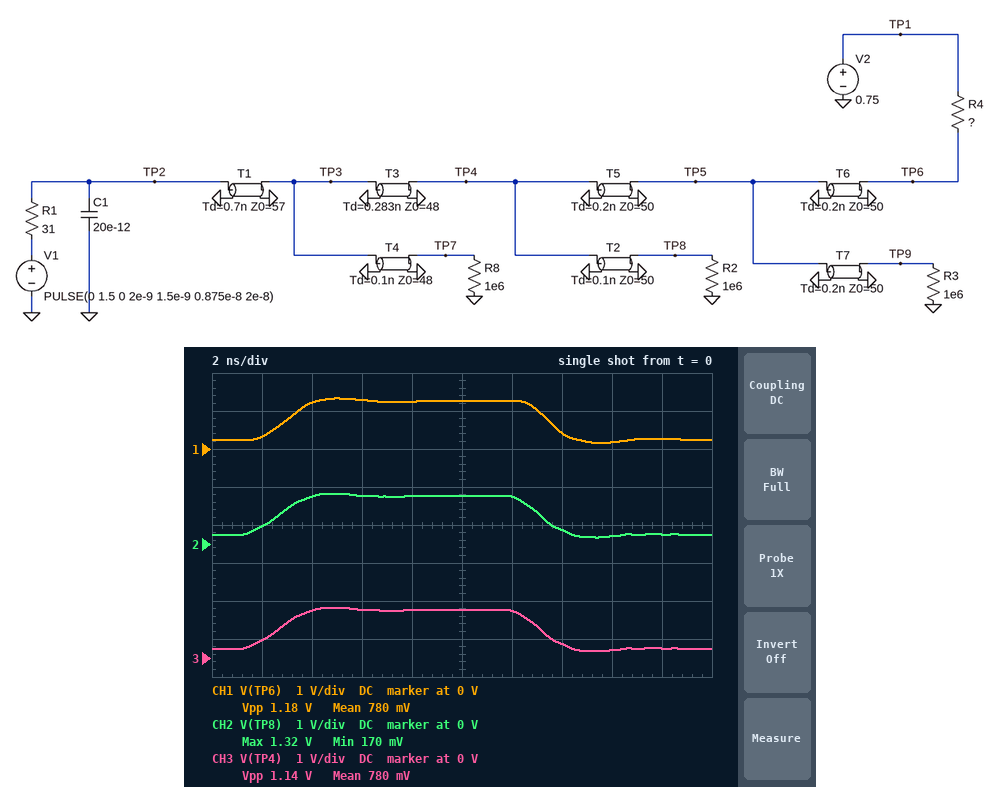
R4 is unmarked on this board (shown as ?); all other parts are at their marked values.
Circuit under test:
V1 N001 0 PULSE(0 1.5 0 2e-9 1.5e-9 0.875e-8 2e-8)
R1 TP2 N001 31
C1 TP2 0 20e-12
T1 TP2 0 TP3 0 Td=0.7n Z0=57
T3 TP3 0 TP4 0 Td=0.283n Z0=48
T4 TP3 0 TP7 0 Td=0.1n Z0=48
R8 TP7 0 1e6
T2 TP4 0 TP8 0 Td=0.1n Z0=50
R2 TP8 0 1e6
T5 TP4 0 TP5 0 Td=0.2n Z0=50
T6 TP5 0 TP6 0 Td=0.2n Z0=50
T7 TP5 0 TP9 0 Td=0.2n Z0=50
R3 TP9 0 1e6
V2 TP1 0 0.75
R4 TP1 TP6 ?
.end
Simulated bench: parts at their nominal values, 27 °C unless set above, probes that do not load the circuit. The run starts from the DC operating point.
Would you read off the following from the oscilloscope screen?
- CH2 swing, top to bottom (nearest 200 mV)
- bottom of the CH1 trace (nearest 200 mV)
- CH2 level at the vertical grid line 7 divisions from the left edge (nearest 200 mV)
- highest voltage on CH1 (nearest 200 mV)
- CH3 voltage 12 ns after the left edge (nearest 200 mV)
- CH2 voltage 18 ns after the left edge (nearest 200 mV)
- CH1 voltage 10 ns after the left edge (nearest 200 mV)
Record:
1.2 V
200 mV
400 mV
1.4 V
1.2 V
200 mV
1.2 V
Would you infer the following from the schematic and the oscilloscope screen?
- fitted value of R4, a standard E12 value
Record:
68 Ω
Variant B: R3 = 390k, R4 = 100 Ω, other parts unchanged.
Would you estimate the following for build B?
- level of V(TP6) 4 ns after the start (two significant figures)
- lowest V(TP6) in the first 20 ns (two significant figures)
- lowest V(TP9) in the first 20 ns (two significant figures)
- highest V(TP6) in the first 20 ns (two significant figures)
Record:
1.3 V
47 mV
46 mV
1.4 V
